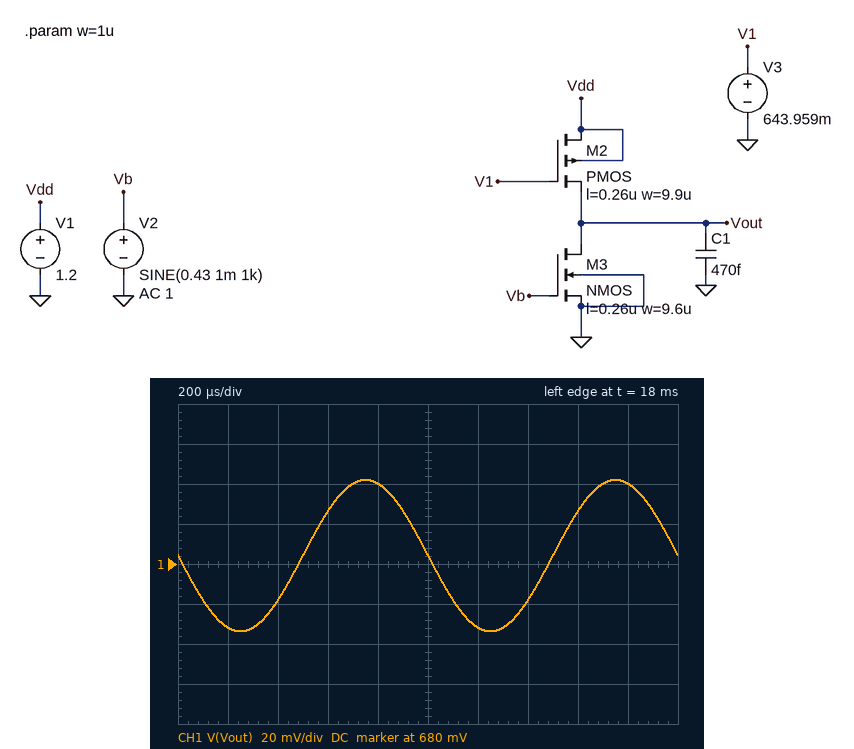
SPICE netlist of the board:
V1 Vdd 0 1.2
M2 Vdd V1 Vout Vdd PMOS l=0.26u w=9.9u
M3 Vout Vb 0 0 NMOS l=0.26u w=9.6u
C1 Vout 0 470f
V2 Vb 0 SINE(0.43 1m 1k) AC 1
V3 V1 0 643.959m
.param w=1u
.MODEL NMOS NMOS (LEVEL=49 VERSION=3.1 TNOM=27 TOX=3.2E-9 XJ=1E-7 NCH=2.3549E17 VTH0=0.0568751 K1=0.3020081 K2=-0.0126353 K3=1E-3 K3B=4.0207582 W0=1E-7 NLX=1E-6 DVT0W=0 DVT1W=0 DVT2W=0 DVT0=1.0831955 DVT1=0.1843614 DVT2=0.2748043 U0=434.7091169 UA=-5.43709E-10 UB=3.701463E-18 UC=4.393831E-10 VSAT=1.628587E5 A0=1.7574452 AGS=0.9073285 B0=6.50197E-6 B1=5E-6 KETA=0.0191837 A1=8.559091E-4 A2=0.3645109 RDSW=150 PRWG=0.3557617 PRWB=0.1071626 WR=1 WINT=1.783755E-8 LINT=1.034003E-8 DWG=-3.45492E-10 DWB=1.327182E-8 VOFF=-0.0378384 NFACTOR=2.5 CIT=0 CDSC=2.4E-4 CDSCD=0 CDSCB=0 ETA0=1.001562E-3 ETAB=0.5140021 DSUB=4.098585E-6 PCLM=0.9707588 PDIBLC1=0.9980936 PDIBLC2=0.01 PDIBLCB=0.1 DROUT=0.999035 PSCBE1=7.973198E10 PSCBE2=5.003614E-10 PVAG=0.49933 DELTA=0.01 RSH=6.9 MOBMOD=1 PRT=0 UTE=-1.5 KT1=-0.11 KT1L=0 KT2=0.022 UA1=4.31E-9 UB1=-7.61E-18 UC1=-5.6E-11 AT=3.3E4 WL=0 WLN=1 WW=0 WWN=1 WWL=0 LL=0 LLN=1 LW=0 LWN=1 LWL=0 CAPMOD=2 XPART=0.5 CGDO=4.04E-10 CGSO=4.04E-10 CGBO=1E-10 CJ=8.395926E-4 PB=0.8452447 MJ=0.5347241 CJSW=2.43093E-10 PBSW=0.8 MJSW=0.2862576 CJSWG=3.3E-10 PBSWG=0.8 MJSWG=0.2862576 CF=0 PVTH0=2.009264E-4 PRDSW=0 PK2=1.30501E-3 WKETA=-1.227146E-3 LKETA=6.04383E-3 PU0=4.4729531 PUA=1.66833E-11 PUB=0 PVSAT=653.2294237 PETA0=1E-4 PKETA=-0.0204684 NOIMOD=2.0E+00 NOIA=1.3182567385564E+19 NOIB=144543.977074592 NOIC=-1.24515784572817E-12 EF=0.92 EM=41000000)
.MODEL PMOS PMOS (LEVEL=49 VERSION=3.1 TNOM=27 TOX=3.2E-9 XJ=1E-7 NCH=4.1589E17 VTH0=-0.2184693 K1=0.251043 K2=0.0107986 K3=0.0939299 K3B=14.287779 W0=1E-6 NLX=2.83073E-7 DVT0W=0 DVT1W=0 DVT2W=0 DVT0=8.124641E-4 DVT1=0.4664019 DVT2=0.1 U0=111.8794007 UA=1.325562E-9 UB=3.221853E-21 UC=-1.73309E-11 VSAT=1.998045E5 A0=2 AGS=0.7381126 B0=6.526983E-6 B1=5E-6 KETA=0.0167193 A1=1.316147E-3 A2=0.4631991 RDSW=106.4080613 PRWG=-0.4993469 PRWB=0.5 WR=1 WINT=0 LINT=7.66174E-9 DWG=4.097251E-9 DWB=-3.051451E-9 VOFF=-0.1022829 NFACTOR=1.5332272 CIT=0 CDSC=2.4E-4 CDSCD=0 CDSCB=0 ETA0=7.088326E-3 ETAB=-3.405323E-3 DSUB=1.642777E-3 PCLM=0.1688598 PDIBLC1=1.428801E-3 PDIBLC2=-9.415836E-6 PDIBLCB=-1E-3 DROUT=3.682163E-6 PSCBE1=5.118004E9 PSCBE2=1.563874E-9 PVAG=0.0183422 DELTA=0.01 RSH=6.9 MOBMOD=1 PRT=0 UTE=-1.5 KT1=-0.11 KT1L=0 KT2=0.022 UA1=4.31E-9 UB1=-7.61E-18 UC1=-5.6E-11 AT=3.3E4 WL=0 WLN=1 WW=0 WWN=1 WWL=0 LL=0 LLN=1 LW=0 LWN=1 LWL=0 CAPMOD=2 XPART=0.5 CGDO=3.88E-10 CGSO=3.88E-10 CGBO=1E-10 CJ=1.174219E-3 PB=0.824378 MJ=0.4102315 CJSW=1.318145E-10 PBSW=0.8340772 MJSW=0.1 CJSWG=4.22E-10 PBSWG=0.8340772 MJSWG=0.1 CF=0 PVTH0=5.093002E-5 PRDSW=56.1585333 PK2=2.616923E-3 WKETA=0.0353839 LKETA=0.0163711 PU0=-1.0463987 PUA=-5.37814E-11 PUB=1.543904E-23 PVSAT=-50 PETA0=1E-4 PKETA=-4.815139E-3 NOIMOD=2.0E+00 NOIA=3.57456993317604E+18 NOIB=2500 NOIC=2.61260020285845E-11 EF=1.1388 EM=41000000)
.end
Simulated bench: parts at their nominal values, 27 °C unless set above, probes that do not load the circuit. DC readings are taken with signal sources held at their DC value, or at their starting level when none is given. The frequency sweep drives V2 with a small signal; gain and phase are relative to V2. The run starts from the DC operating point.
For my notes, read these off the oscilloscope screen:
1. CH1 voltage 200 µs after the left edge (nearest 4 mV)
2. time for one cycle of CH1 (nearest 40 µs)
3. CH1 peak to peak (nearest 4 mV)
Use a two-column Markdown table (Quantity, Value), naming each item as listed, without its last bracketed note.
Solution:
| Quantity | Value |
|---|---|
| CH1 voltage 200 µs after the left edge | 648 mV |
| time for one cycle of CH1 | 1.00 ms |
| CH1 peak to peak | 76 mV |
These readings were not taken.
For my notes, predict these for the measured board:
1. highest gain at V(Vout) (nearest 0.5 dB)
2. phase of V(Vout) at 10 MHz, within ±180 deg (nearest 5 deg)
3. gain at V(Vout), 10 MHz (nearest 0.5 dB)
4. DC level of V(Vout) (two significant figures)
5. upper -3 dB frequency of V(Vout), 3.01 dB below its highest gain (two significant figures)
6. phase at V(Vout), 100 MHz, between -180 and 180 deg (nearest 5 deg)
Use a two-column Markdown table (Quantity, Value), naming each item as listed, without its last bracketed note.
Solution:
| Quantity | Value |
|---|---|
| highest gain at V(Vout) | 31.5 dB |
| phase of V(Vout) at 10 MHz, within ±180 deg | 145 deg |
| gain at V(Vout), 10 MHz | 30.0 dB |
| DC level of V(Vout) | 680 mV |
| upper -3 dB frequency of V(Vout), 3.01 dB below its highest gain | 15 MHz |
| phase at V(Vout), 100 MHz, between -180 and 180 deg | 100 deg |
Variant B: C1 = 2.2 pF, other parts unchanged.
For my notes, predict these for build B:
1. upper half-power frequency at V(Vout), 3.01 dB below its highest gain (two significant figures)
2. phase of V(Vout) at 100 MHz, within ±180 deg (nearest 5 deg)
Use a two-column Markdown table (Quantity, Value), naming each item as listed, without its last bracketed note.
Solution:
| Quantity | Value |
|---|---|
| upper half-power frequency at V(Vout), 3.01 dB below its highest gain | 3.2 MHz |
| phase of V(Vout) at 100 MHz, within ±180 deg | 90 deg |
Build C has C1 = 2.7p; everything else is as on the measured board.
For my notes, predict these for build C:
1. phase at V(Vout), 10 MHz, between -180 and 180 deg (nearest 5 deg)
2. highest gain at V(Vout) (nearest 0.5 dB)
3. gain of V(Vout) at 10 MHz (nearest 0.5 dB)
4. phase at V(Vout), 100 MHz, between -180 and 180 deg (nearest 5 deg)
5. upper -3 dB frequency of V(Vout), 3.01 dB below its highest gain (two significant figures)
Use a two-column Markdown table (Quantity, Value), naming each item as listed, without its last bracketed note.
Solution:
| Quantity | Value |
|---|---|
| phase at V(Vout), 10 MHz, between -180 and 180 deg | 105 deg |
| highest gain at V(Vout) | 31.5 dB |
| gain of V(Vout) at 10 MHz | 19.5 dB |
| phase at V(Vout), 100 MHz, between -180 and 180 deg | 90 deg |
| upper -3 dB frequency of V(Vout), 3.01 dB below its highest gain | 2.6 MHz |
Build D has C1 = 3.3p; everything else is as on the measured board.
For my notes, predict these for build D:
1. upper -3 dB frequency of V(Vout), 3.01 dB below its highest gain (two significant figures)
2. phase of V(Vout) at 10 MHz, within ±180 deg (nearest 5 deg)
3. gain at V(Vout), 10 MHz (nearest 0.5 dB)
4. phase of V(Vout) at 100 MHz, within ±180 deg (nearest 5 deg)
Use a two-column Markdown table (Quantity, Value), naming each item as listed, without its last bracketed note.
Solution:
| Quantity | Value |
|---|---|
| upper -3 dB frequency of V(Vout), 3.01 dB below its highest gain | 2.1 MHz |
| phase of V(Vout) at 10 MHz, within ±180 deg | 100 deg |
| gain at V(Vout), 10 MHz | 18.0 dB |
| phase of V(Vout) at 100 MHz, within ±180 deg | 90 deg |
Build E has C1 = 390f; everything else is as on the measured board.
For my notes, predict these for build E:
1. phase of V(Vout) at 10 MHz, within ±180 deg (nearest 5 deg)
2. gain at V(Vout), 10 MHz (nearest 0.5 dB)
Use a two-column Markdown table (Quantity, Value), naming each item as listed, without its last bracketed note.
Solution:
| Quantity | Value |
|---|---|
| phase of V(Vout) at 10 MHz, within ±180 deg | 150 deg |
| gain at V(Vout), 10 MHz | 30.5 dB |
